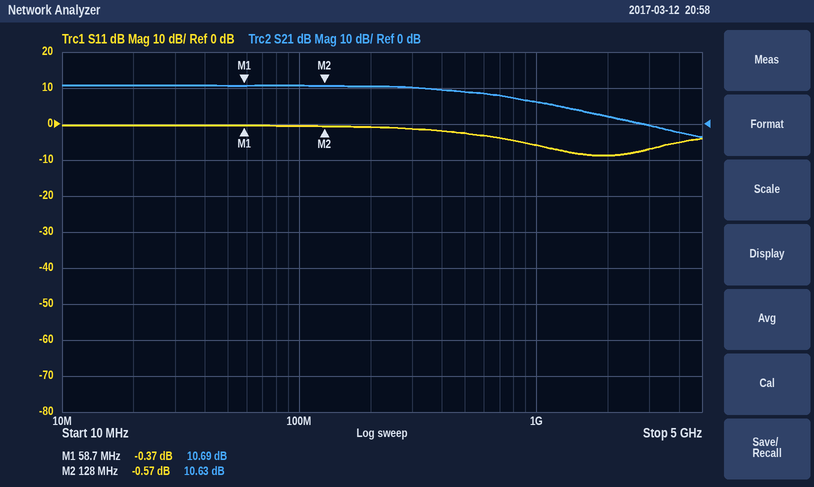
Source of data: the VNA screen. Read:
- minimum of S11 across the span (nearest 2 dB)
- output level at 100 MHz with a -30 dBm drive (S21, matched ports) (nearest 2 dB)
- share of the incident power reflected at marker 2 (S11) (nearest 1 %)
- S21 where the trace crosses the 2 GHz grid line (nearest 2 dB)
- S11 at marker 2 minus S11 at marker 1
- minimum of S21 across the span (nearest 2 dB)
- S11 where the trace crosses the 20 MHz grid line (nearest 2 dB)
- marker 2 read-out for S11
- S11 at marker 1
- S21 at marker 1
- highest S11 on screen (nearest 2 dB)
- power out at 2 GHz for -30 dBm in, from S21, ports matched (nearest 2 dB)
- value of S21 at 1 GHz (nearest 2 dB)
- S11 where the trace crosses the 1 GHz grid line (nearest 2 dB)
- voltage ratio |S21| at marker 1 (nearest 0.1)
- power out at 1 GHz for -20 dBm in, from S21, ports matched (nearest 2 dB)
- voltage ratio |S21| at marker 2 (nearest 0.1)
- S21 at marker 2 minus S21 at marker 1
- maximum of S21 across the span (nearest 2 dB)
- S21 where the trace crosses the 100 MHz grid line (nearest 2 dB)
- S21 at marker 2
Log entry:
-8 dB
-20 dBm
88 %
2 dB
-0.20 dB
-4 dB
0 dB
-0.57 dB
-0.37 dB
10.69 dB
0 dB
-28 dBm
6 dB
-6 dB
3.4
-14 dBm
3.4
-0.06 dB
10 dB
10 dB
10.63 dB
